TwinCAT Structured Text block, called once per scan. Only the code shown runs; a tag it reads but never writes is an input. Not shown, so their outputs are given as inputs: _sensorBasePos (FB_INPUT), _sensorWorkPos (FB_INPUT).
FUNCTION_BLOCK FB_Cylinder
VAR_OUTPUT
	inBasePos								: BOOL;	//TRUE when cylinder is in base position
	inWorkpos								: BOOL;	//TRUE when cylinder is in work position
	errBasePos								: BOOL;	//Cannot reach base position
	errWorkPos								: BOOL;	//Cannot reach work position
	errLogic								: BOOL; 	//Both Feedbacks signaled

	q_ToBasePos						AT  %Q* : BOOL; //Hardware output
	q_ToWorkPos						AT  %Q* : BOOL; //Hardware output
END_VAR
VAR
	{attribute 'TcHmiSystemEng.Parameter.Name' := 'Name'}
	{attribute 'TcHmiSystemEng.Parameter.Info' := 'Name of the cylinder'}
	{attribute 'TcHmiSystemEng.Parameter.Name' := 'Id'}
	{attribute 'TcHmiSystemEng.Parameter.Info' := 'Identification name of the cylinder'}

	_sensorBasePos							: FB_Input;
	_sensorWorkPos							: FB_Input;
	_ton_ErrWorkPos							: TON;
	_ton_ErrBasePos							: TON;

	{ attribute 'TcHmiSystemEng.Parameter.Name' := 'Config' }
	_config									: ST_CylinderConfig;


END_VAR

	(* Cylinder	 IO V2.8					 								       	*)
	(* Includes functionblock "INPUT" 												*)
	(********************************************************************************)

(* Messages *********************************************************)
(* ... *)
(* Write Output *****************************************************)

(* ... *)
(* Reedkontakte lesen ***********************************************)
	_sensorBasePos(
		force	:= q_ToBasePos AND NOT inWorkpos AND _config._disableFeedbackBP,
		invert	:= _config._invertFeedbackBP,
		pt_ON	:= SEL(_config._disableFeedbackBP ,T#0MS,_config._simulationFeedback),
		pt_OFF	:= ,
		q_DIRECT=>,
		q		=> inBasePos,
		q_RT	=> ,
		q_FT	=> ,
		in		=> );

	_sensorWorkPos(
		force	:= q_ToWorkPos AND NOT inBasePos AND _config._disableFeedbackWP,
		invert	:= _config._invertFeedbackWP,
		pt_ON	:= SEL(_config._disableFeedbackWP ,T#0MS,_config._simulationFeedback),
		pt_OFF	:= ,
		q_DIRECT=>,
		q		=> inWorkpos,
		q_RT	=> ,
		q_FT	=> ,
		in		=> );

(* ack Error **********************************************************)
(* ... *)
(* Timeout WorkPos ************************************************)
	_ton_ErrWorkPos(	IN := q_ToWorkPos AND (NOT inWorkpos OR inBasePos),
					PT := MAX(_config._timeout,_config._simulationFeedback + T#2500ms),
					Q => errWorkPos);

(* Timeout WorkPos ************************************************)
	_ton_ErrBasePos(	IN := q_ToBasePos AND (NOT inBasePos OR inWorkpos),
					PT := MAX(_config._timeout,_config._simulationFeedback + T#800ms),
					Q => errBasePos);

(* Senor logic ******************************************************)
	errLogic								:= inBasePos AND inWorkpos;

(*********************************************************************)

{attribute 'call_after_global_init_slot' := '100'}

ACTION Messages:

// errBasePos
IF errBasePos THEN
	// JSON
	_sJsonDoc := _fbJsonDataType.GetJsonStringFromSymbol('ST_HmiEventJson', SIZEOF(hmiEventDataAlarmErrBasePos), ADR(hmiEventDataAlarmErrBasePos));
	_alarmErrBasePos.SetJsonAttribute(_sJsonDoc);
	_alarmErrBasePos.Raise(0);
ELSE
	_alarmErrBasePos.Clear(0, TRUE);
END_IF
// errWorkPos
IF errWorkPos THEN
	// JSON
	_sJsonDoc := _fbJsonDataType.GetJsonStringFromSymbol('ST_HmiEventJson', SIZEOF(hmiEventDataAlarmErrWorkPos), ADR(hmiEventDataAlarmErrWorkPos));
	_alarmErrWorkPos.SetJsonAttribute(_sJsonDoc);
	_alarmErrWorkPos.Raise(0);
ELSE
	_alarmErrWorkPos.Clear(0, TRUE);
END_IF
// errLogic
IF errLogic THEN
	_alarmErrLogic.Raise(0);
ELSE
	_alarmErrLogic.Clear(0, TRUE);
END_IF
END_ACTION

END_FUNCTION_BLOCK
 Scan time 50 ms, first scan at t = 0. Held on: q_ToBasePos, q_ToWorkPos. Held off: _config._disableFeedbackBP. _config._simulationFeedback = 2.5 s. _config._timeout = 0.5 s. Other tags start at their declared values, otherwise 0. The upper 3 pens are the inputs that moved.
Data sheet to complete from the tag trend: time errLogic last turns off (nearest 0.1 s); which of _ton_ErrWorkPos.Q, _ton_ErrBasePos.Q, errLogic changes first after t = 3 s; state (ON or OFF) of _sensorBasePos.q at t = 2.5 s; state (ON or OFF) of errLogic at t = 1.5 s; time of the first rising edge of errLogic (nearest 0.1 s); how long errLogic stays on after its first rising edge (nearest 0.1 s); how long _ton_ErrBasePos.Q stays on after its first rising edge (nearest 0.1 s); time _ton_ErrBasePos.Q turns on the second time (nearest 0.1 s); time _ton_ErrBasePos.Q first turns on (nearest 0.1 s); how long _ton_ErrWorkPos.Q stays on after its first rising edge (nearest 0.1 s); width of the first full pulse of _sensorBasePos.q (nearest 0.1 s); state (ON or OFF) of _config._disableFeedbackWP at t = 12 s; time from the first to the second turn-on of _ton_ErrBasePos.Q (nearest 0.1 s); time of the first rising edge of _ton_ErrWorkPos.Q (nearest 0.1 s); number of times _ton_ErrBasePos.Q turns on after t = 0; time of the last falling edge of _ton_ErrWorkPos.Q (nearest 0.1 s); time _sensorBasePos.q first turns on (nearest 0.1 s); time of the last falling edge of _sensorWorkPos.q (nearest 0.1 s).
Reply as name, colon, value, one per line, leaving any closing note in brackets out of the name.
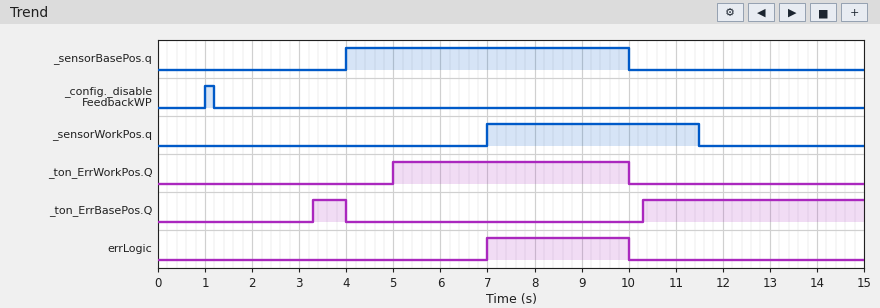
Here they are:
time errLogic last turns off: 10.0 s
which of _ton_ErrWorkPos.Q, _ton_ErrBasePos.Q, errLogic changes first after t = 3 s: _ton_ErrBasePos.Q
state (ON or OFF) of _sensorBasePos.q at t = 2.5 s: OFF
state (ON or OFF) of errLogic at t = 1.5 s: OFF
time of the first rising edge of errLogic: 7.0 s
how long errLogic stays on after its first rising edge: 3.0 s
how long _ton_ErrBasePos.Q stays on after its first rising edge: 0.7 s
time _ton_ErrBasePos.Q turns on the second time: 10.3 s
time _ton_ErrBasePos.Q first turns on: 3.3 s
how long _ton_ErrWorkPos.Q stays on after its first rising edge: 5.0 s
width of the first full pulse of _sensorBasePos.q: 6.0 s
state (ON or OFF) of _config._disableFeedbackWP at t = 12 s: OFF
time from the first to the second turn-on of _ton_ErrBasePos.Q: 7.0 s
time of the first rising edge of _ton_ErrWorkPos.Q: 5.0 s
number of times _ton_ErrBasePos.Q turns on after t = 0: 2
time of the last falling edge of _ton_ErrWorkPos.Q: 10.0 s
time _sensorBasePos.q first turns on: 4.0 s
time of the last falling edge of _sensorWorkPos.q: 11.5 s
